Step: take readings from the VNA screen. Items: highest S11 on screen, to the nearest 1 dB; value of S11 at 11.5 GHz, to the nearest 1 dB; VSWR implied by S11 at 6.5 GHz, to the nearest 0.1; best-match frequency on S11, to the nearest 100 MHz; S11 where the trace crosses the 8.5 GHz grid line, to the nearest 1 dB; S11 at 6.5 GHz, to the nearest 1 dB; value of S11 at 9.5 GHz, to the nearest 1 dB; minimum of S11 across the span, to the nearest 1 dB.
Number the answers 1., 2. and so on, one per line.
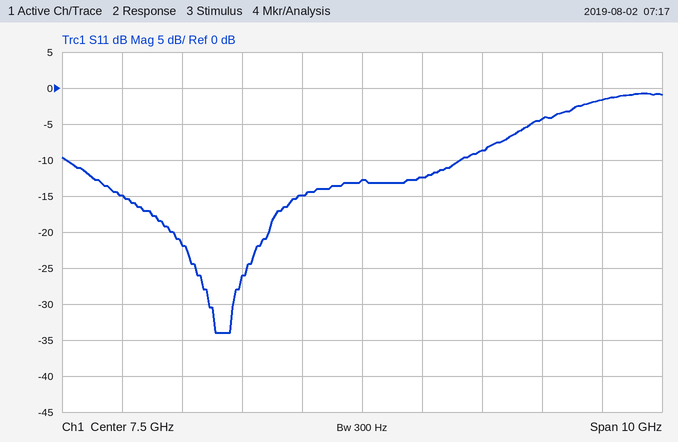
1. -1 dB
2. -2 dB
3. 1.4
4. 5.1 GHz
5. -12 dB
6. -15 dB
7. -9 dB
8. -34 dB
